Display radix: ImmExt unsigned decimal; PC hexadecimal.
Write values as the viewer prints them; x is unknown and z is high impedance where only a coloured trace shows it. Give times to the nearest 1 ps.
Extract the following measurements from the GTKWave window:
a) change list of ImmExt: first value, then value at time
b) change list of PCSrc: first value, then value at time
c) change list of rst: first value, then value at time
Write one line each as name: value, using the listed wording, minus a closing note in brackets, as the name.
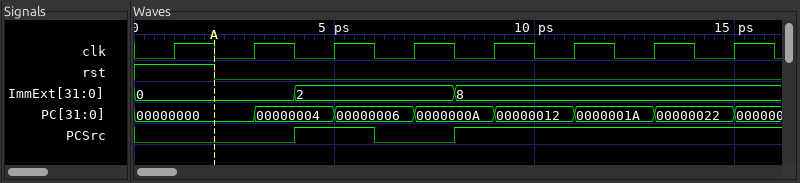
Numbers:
change list of ImmExt: first value, then value at time: 0, 2 at 4 ps, 8 at 8 ps
change list of PCSrc: first value, then value at time: 0, 1 at 4 ps, 0 at 6 ps, 1 at 8 ps
change list of rst: first value, then value at time: 1, 0 at 2 ps
